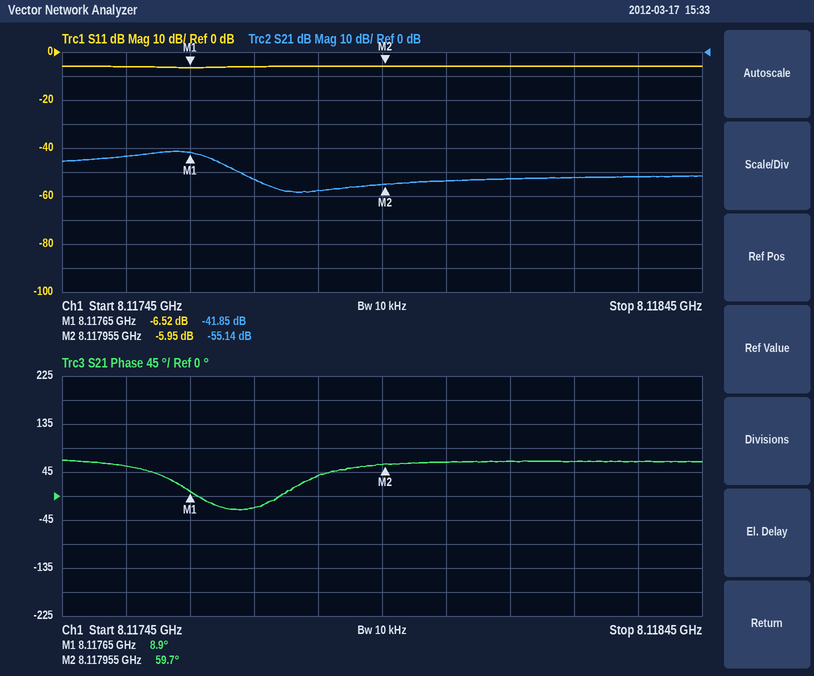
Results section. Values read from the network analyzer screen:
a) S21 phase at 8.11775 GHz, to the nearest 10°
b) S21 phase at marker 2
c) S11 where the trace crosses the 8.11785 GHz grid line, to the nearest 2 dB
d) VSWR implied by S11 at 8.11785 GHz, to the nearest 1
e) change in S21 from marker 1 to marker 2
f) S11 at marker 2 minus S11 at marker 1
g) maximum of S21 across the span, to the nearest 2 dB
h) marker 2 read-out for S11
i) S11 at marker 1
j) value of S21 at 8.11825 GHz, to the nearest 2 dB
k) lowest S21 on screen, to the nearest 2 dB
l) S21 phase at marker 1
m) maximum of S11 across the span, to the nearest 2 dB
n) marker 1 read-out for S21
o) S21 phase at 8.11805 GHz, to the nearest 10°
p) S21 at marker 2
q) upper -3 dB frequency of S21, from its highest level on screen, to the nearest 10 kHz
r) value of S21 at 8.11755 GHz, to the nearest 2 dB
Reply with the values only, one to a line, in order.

-20°
59.7°
-6 dB
3
-13.29 dB
0.57 dB
-42 dB
-5.95 dB
-6.52 dB
-52 dB
-58 dB
8.9°
-6 dB
-41.85 dB
60°
-55.14 dB
8.11768 GHz
-44 dB
